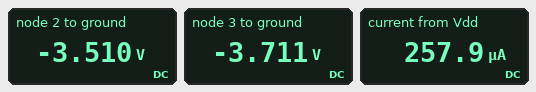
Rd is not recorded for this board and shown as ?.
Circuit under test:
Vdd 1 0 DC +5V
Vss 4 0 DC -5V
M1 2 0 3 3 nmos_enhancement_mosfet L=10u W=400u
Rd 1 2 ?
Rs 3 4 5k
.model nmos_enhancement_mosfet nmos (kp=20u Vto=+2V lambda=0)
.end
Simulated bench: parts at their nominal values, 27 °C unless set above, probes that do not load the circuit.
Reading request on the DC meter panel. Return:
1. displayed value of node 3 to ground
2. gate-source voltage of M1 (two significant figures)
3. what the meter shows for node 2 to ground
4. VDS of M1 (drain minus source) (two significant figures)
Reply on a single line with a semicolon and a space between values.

-3.711 V; 3.7 V; -3.510 V; 200 mV
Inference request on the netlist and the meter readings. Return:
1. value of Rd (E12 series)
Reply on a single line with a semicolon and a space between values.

33 kΩ
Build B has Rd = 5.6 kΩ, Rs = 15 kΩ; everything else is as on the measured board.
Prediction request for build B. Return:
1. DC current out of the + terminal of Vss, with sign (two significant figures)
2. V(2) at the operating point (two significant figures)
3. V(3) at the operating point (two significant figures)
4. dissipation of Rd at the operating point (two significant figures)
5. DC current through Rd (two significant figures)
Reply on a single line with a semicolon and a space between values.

-160 µA; 4.1 V; -2.6 V; 140 µW; 160 µA
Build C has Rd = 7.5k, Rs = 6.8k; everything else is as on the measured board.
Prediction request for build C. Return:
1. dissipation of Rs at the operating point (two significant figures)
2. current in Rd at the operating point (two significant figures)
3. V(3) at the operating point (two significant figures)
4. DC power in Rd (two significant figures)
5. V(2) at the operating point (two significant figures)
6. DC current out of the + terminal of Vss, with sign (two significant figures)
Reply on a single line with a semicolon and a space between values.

660 µW; 310 µA; -2.9 V; 730 µW; 2.7 V; -310 µA
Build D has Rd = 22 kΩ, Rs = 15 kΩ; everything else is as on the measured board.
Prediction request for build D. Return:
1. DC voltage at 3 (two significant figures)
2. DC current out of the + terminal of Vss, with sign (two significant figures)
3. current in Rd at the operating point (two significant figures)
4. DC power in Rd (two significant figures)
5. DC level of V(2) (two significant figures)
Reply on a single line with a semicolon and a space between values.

-2.6 V; -160 µA; 160 µA; 550 µW; 1.5 V
